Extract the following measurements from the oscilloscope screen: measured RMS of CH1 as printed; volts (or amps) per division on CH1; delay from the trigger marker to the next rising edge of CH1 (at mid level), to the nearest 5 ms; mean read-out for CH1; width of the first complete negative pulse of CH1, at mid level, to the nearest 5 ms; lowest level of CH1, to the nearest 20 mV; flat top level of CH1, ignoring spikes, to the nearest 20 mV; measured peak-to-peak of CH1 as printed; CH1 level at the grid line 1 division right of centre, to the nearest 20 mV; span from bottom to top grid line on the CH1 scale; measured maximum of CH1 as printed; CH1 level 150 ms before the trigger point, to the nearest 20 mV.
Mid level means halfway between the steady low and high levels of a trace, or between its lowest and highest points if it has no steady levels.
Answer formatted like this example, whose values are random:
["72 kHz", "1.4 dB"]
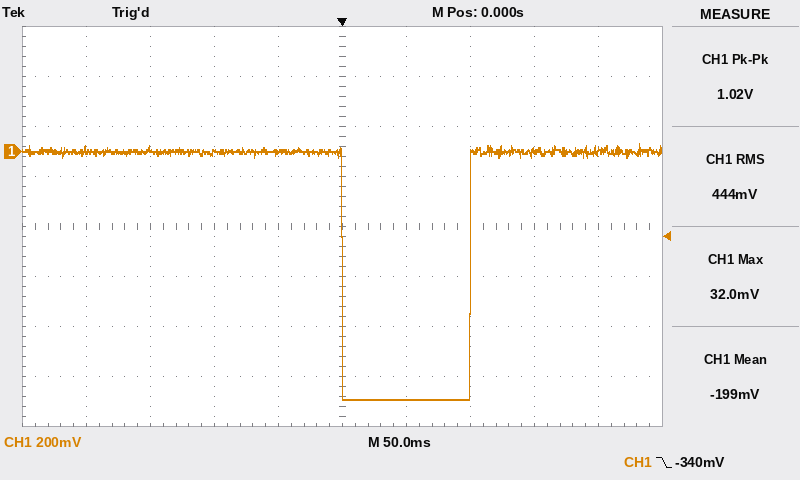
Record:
["444 mV", "200 mV", "100 ms", "-199 mV", "100 ms", "-1.00 V", "0 mV", "1.02 V", "-1.00 V", "1.6 V", "32.0 mV", "20 mV"]
